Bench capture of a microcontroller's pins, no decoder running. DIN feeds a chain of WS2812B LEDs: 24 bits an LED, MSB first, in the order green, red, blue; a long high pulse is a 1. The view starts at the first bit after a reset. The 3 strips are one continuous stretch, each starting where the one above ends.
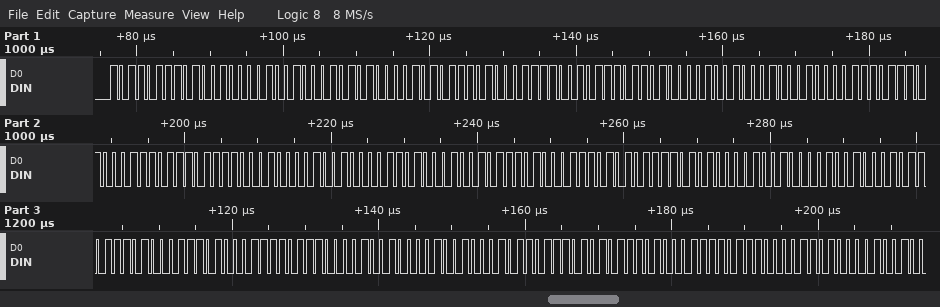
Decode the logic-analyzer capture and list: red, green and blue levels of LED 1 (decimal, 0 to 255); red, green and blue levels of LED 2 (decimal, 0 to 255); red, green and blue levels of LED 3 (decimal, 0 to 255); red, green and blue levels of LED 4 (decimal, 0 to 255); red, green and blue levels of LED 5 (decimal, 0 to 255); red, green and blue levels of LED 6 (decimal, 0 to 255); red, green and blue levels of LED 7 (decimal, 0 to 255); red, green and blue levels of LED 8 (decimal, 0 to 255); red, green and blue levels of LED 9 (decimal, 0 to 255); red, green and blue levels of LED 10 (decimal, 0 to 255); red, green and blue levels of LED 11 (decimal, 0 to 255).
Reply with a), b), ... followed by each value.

a) 72, 183, 72
b) 87, 168, 71
c) 104, 151, 72
d) 119, 136, 71
e) 136, 119, 72
f) 151, 104, 71
g) 168, 87, 72
h) 183, 72, 71
i) 184, 71, 72
j) 183, 72, 87
k) 184, 71, 104
